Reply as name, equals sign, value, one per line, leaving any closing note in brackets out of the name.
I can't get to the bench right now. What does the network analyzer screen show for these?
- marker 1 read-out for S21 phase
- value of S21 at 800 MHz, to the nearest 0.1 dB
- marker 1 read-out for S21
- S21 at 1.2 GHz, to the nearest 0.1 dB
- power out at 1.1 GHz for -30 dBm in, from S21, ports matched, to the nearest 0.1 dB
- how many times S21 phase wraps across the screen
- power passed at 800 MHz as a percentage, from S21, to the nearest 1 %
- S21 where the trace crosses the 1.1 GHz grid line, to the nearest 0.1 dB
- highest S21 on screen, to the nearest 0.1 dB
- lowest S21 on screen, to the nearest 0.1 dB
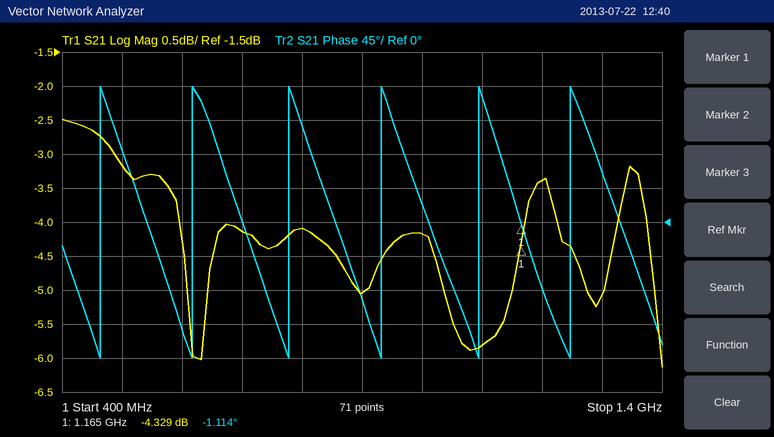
marker 1 read-out for S21 phase = -1.114°
value of S21 at 800 MHz, to the nearest 0.1 dB = -4.1 dB
marker 1 read-out for S21 = -4.329 dB
S21 at 1.2 GHz, to the nearest 0.1 dB = -3.4 dB
power out at 1.1 GHz for -30 dBm in, from S21, ports matched, to the nearest 0.1 dB = -35.8 dBm
how many times S21 phase wraps across the screen = 6
power passed at 800 MHz as a percentage, from S21, to the nearest 1 % = 39 %
S21 where the trace crosses the 1.1 GHz grid line, to the nearest 0.1 dB = -5.8 dB
highest S21 on screen, to the nearest 0.1 dB = -2.5 dB
lowest S21 on screen, to the nearest 0.1 dB = -6.1 dB
